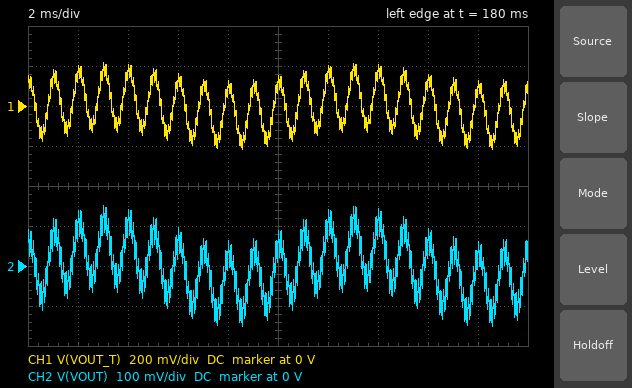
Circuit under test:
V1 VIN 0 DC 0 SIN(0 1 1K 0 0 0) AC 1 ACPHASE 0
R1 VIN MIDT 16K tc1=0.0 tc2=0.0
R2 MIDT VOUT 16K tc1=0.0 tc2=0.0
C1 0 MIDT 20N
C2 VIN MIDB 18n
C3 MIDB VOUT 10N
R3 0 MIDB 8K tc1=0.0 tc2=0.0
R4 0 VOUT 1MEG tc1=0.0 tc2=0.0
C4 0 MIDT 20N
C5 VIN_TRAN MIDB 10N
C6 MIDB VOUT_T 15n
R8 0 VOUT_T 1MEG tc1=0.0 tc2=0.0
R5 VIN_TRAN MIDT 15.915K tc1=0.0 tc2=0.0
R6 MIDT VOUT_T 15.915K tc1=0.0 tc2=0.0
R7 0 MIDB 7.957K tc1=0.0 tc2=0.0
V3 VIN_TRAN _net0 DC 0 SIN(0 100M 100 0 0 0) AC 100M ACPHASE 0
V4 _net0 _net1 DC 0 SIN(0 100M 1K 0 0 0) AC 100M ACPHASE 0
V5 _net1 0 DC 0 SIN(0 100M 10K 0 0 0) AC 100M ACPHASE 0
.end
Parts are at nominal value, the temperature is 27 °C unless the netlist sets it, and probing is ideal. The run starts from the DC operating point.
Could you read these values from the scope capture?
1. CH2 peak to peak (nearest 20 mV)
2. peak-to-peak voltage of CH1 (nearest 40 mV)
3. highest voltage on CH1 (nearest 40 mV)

300 mV
440 mV
200 mV
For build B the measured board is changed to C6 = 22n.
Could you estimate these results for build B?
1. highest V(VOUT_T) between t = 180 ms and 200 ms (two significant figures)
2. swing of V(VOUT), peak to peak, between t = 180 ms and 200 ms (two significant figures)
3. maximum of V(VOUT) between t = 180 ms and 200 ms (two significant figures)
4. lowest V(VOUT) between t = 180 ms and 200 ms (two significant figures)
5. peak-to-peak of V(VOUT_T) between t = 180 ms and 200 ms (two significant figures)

250 mV
280 mV
140 mV
-140 mV
510 mV
